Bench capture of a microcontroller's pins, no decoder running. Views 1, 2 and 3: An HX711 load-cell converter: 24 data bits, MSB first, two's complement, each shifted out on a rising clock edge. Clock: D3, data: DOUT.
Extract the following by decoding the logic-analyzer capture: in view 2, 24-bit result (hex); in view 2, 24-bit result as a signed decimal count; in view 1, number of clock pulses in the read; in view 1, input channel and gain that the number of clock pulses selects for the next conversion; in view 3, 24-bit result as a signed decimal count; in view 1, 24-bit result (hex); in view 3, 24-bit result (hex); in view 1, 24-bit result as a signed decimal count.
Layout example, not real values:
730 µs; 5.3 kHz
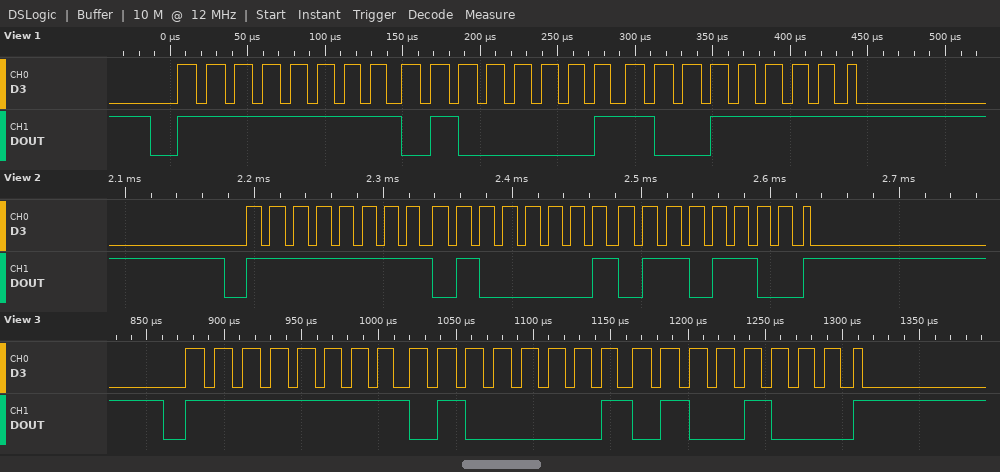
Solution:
0xFF416C; -48788; 25; channel A, gain 128; -48824; 0xFF419F; 0xFF4148; -48737
